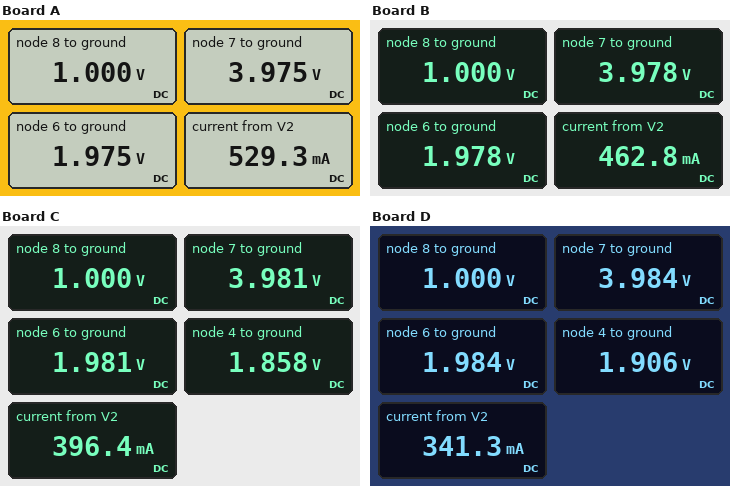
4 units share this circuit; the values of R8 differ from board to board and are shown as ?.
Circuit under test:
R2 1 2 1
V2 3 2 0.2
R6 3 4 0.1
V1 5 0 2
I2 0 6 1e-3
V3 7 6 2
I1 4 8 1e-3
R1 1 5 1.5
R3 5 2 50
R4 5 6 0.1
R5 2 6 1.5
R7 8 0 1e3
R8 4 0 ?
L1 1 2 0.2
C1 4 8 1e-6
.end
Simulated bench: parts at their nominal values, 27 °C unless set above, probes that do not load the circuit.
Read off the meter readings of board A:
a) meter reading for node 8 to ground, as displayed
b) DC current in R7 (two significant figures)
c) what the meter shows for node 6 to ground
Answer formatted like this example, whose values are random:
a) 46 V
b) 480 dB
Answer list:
a) 1.000 V
b) 1.0 mA
c) 1.975 V
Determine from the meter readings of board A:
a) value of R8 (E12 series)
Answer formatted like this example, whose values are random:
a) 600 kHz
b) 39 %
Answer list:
a) 3.3 Ω
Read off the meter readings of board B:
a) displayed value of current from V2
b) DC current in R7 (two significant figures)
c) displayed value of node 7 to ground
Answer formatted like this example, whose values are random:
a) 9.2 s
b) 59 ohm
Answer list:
a) 462.8 mA
b) 1.0 mA
c) 3.978 V
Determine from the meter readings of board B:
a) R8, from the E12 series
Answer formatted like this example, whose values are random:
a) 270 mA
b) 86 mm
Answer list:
a) 3.9 Ω
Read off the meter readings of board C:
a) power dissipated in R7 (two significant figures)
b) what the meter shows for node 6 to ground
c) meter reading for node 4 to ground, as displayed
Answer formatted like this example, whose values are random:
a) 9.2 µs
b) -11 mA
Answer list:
a) 1.0 mW
b) 1.981 V
c) 1.858 V
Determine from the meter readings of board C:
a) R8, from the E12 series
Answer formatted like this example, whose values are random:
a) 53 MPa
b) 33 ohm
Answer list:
a) 4.7 Ω
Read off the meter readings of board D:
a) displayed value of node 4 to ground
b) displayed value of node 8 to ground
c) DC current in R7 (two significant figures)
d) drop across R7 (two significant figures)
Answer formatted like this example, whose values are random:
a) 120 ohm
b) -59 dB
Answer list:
a) 1.906 V
b) 1.000 V
c) 1.0 mA
d) 1.0 V
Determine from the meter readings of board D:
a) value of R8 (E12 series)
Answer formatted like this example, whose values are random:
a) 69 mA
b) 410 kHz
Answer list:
a) 5.6 Ω
